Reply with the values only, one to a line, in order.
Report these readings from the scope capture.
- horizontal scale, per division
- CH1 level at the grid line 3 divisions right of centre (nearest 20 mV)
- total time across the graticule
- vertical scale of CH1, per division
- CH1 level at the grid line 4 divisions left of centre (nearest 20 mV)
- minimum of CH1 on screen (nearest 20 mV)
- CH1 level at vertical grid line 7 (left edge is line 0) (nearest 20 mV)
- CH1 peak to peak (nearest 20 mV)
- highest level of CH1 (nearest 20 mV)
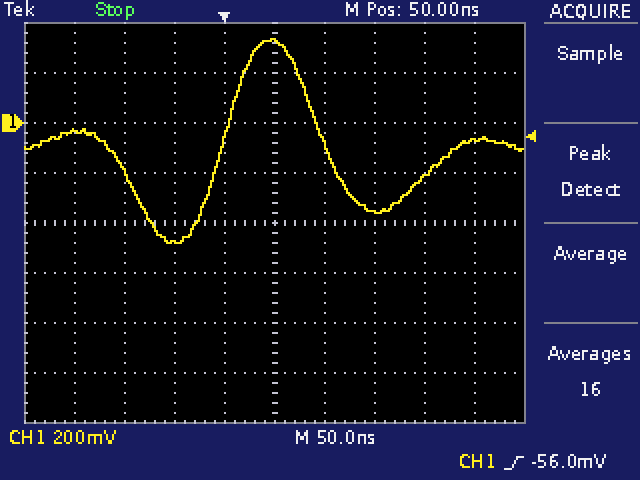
50 ns
-220 mV
500 ns
200 mV
-40 mV
-480 mV
-360 mV
820 mV
340 mV
